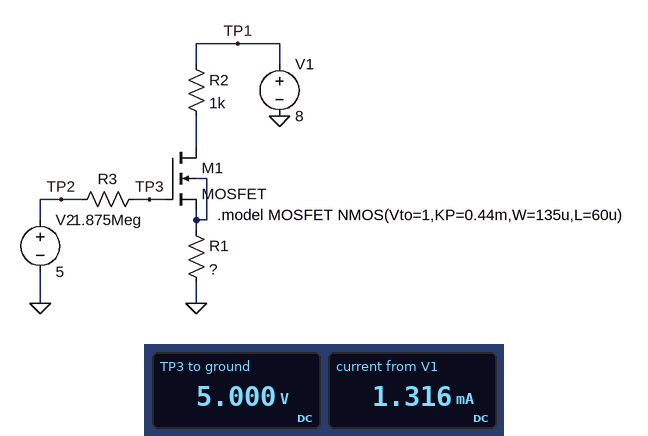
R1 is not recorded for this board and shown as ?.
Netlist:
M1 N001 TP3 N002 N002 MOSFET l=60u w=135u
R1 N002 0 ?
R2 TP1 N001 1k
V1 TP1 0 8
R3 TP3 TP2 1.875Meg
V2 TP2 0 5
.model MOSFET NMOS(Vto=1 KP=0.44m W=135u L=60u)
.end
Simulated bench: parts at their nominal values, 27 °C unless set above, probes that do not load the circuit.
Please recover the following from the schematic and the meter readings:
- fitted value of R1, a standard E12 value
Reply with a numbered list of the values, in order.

1. 1.8 kΩ
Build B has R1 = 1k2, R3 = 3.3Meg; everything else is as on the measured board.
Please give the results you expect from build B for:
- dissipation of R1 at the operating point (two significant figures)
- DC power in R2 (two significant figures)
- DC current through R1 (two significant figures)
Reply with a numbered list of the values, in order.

1. 3.7 mW
2. 3.1 mW
3. 1.8 mA
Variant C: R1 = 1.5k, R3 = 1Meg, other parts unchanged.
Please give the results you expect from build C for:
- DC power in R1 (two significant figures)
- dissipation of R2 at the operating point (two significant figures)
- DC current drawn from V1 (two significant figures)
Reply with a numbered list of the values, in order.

1. 3.4 mW
2. 2.3 mW
3. 1.5 mA
